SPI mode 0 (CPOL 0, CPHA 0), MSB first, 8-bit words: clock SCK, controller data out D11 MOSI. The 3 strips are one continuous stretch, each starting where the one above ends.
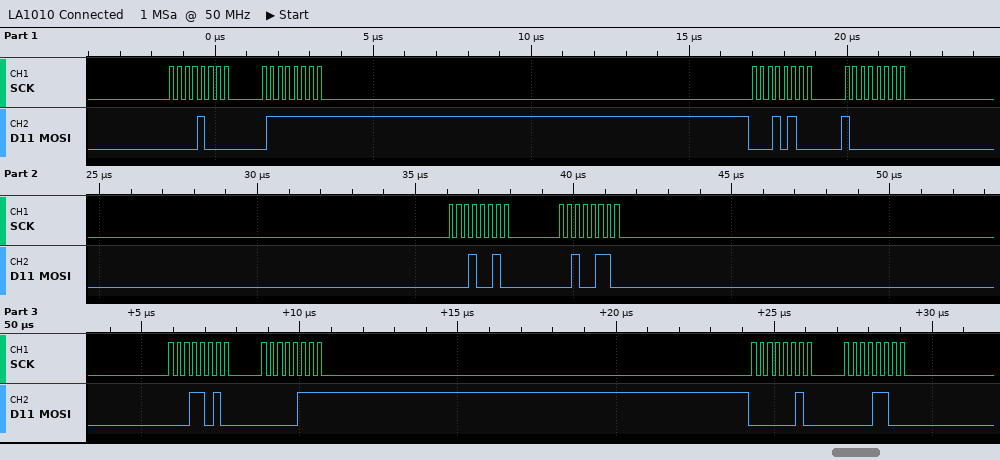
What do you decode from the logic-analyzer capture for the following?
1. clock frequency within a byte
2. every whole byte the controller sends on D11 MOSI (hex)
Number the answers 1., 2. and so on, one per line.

1. 4 MHz
2. 08 7F 14 80 12 26 1A 07 02 0C
